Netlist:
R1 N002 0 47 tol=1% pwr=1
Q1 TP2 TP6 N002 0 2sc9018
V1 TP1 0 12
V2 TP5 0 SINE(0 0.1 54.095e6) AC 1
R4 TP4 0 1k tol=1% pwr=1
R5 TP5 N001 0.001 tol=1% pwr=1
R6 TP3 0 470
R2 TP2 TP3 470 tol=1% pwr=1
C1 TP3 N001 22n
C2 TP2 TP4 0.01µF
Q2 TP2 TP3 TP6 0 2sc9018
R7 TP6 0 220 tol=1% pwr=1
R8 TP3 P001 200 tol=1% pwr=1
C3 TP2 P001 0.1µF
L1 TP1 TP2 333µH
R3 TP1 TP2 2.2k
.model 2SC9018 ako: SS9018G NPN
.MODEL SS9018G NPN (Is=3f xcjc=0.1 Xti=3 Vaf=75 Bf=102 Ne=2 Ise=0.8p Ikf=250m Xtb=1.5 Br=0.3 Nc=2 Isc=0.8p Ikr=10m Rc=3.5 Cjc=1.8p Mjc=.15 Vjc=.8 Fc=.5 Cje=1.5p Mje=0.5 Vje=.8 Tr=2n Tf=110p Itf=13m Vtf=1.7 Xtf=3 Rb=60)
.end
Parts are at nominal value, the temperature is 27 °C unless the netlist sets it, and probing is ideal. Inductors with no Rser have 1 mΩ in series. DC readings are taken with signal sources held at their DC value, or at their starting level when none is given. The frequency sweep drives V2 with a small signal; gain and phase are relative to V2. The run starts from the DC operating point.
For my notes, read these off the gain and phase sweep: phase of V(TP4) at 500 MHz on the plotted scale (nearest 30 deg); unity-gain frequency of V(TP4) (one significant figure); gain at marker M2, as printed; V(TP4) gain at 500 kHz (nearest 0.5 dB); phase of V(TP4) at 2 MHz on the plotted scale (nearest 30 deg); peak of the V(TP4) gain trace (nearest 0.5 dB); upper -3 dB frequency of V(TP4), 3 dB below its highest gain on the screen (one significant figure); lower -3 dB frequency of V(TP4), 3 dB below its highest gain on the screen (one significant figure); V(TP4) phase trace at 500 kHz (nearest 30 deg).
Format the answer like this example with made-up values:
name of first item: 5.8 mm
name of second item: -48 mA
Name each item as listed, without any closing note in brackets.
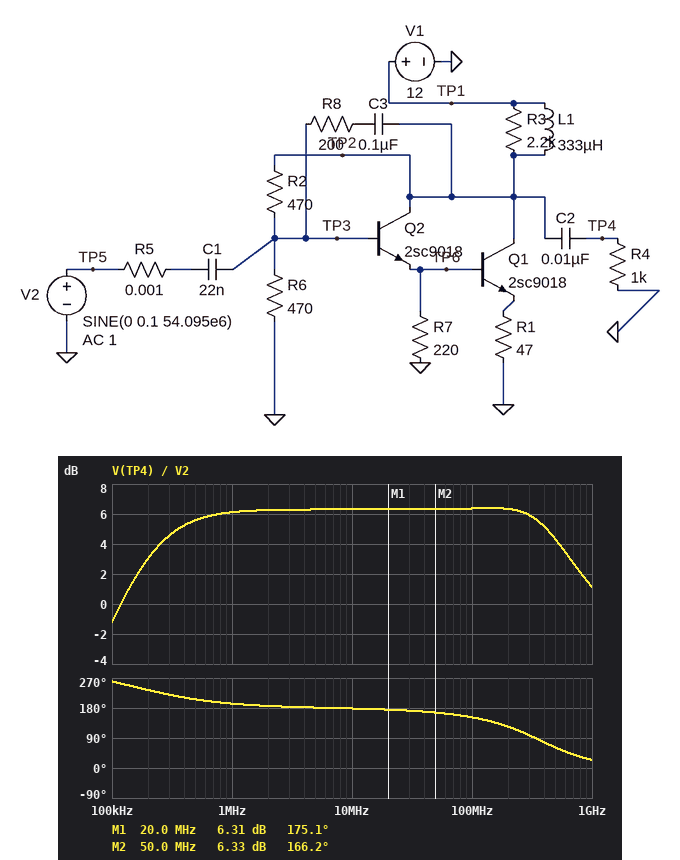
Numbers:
phase of V(TP4) at 500 MHz on the plotted scale: 60 deg
unity-gain frequency of V(TP4): 100 kHz
gain at marker M2, as printed: 6.33 dB
V(TP4) gain at 500 kHz: 5.5 dB
phase of V(TP4) at 2 MHz on the plotted scale: 180 deg
peak of the V(TP4) gain trace: 6.5 dB
upper -3 dB frequency of V(TP4), 3 dB below its highest gain on the screen: 600 MHz
lower -3 dB frequency of V(TP4), 3 dB below its highest gain on the screen: 200 kHz
V(TP4) phase trace at 500 kHz: 210 deg
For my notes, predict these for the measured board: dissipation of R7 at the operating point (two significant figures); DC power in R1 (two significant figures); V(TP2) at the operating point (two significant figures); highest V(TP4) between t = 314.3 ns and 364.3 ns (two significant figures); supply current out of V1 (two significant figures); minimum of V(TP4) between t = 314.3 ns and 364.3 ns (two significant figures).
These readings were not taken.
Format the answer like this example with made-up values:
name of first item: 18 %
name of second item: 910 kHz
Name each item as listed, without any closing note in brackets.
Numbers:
dissipation of R7 at the operating point: 120 mW
DC power in R1: 390 mW
V(TP2) at the operating point: 12 V
highest V(TP4) between t = 314.3 ns and 364.3 ns: 210 mV
supply current out of V1: 130 mA
minimum of V(TP4) between t = 314.3 ns and 364.3 ns: -210 mV
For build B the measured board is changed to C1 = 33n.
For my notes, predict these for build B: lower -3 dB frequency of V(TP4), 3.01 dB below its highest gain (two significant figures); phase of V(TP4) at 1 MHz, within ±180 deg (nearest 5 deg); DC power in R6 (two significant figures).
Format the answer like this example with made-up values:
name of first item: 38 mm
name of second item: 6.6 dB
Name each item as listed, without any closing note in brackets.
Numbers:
lower -3 dB frequency of V(TP4), 3.01 dB below its highest gain: 160 kHz
phase of V(TP4) at 1 MHz, within ±180 deg: -170 deg
DC power in R6: 75 mW
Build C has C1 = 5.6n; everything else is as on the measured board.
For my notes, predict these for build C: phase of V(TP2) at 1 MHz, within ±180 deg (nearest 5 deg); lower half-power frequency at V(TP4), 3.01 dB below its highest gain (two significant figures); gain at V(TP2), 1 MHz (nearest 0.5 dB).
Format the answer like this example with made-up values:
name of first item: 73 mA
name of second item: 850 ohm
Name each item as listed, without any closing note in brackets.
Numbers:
phase of V(TP2) at 1 MHz, within ±180 deg: -145 deg
lower half-power frequency at V(TP4), 3.01 dB below its highest gain: 730 kHz
gain at V(TP2), 1 MHz: 4.5 dB
